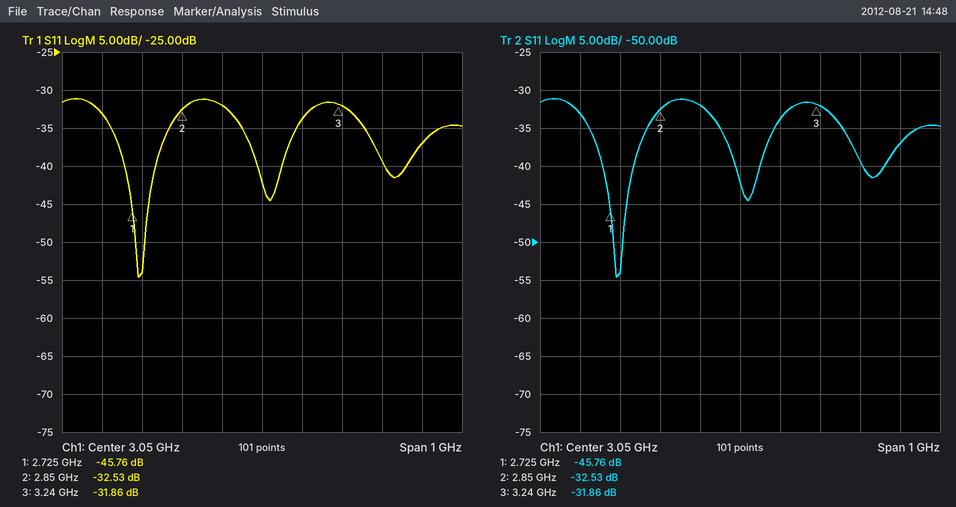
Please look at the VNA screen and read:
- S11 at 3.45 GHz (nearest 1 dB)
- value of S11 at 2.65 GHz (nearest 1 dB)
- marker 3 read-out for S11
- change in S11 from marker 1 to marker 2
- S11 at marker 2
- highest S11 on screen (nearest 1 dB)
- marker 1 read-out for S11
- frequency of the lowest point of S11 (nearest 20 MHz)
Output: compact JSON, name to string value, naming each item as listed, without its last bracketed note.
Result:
{"S11 at 3.45 GHz": "-37 dB", "value of S11 at 2.65 GHz": "-33 dB", "marker 3 read-out for S11": "-31.86 dB", "change in S11 from marker 1 to marker 2": "13.23 dB", "S11 at marker 2": "-32.53 dB", "highest S11 on screen": "-31 dB", "marker 1 read-out for S11": "-45.76 dB", "frequency of the lowest point of S11": "2.74 GHz"}
